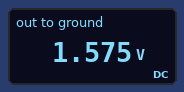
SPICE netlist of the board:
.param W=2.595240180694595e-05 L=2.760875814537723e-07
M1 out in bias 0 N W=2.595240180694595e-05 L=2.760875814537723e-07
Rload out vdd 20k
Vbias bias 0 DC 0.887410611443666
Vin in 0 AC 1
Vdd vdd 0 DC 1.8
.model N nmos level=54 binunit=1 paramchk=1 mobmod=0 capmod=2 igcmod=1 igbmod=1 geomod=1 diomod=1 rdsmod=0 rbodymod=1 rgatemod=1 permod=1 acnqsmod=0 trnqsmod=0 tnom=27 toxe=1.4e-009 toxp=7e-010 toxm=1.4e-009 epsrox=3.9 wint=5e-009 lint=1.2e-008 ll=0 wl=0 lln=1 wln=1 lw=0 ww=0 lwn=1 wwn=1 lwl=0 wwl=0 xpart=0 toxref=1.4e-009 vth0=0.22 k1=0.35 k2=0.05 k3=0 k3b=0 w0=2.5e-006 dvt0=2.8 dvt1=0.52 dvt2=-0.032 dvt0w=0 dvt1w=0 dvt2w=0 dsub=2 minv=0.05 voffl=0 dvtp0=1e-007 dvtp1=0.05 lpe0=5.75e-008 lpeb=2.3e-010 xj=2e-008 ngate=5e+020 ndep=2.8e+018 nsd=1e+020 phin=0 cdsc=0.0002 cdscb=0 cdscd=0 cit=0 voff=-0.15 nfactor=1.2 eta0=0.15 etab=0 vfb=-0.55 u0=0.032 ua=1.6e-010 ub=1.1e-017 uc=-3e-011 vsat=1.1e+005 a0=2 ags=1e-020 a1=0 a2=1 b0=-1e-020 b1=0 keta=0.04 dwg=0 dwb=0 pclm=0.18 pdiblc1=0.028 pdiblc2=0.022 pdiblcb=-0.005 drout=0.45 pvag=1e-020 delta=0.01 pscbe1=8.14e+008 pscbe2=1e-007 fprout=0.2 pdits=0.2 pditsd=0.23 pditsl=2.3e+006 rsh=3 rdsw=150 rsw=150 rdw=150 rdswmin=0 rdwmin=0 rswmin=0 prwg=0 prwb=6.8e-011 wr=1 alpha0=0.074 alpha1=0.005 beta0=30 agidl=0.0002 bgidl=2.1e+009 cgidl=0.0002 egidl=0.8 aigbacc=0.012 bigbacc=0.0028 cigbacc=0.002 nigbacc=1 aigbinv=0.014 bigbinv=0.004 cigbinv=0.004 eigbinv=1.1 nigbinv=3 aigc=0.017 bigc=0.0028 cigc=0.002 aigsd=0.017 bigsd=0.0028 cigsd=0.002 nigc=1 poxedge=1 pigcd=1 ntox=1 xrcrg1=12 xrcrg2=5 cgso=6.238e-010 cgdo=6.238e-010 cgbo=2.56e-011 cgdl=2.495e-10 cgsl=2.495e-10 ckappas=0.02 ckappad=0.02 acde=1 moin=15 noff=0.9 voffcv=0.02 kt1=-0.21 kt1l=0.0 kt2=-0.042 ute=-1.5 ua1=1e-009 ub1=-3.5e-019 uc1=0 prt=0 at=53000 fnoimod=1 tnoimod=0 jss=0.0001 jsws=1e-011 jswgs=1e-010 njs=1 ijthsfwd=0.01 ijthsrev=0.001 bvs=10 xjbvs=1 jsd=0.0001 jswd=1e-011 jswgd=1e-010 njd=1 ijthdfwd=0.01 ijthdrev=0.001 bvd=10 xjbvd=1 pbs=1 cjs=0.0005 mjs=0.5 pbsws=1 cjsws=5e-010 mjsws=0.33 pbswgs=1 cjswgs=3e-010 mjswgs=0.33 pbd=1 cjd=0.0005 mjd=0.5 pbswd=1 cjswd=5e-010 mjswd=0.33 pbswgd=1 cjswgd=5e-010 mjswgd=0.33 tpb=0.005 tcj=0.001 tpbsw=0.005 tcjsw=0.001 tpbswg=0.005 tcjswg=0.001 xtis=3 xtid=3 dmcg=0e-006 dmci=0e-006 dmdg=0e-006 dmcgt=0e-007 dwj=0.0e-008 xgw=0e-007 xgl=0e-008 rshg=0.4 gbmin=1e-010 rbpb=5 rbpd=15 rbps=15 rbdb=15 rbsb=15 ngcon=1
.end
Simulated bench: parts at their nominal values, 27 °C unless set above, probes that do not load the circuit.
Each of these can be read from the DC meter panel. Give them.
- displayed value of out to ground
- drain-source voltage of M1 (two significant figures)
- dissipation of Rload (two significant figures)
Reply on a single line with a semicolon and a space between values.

1.575 V; 690 mV; 2.5 µW
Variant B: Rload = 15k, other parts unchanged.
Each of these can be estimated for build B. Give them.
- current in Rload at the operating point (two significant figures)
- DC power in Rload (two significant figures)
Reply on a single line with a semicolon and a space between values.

14 µA; 3.0 µW
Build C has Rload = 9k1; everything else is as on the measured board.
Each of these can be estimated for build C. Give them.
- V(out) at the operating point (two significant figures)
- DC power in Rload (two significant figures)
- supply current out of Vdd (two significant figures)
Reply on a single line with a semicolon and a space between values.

1.6 V; 3.8 µW; 20 µA
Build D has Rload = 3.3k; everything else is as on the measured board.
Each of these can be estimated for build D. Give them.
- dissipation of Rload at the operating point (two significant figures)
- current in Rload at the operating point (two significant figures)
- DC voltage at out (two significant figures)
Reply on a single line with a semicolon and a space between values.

5.5 µW; 41 µA; 1.7 V
